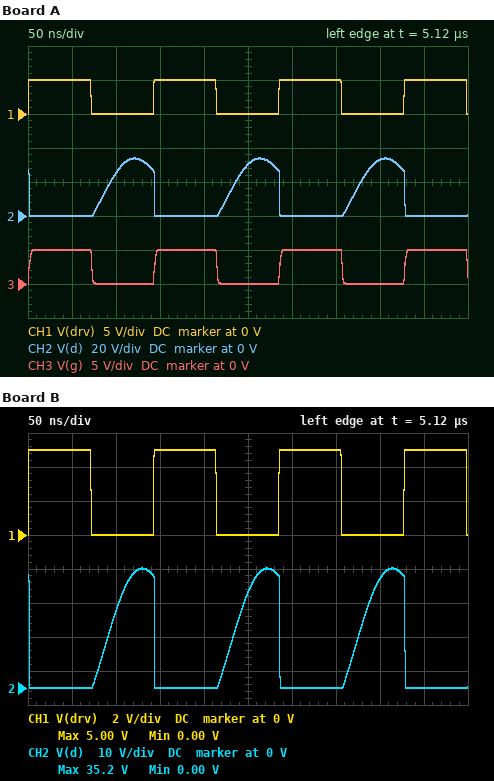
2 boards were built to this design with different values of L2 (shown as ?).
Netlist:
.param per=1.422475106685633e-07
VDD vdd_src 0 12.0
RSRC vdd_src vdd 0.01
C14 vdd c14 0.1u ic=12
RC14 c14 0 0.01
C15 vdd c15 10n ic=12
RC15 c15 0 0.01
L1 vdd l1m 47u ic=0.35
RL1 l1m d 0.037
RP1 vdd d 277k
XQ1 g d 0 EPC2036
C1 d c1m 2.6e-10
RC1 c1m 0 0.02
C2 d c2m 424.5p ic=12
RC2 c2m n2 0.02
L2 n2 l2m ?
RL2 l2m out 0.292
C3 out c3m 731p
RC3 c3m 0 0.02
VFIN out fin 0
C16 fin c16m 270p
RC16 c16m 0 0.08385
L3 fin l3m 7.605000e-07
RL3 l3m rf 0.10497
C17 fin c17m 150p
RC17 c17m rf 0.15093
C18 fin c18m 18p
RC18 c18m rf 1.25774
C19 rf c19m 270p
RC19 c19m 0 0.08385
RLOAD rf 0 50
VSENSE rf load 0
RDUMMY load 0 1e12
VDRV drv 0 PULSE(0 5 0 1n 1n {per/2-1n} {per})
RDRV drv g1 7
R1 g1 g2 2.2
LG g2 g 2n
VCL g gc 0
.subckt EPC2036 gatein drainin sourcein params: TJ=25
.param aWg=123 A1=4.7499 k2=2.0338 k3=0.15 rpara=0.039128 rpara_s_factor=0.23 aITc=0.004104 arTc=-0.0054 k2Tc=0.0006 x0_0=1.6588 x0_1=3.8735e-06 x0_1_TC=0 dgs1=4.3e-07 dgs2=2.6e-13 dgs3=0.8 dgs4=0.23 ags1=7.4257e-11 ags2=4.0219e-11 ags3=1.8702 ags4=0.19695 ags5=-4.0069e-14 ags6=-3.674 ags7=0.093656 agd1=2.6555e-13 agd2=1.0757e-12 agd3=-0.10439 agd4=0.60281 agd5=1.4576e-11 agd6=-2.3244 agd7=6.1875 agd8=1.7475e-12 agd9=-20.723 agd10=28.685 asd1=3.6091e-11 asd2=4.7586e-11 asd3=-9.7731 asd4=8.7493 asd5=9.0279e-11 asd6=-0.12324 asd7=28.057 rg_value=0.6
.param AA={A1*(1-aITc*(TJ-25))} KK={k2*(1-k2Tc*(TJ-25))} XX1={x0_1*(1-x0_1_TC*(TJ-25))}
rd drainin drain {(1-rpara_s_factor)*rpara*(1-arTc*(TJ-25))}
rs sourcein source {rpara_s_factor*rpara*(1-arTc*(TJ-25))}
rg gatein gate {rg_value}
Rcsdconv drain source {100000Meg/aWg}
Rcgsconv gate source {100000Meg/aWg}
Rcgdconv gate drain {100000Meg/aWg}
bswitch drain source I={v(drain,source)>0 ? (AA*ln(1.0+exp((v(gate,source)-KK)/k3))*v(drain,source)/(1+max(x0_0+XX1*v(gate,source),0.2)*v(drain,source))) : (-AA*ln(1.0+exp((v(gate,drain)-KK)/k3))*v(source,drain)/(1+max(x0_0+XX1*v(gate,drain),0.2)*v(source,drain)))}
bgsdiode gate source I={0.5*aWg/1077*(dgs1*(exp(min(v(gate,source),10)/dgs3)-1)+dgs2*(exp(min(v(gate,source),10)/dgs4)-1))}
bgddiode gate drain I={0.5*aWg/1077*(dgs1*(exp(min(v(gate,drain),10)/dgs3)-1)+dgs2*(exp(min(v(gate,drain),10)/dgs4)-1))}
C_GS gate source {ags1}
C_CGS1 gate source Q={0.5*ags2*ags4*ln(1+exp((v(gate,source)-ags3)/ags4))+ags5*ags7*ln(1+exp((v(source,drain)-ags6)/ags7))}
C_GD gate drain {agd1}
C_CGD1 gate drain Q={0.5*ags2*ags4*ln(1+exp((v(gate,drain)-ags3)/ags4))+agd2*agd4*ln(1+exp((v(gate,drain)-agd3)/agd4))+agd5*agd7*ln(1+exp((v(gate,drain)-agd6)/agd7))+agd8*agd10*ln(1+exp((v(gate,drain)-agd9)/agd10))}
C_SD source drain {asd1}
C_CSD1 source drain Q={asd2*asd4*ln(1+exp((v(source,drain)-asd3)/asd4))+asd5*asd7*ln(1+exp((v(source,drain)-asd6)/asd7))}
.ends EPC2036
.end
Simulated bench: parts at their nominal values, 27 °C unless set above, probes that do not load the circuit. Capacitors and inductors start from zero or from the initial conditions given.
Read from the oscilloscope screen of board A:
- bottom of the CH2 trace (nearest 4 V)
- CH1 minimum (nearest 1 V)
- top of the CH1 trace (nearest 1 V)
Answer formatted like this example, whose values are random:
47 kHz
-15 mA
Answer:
0 V
0 V
5 V
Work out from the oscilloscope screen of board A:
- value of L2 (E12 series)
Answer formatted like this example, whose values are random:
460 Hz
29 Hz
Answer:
3.3 µH
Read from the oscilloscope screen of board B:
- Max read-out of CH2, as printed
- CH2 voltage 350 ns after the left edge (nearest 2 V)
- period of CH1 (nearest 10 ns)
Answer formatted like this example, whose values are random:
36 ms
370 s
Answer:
35.2 V
0 V
140 ns
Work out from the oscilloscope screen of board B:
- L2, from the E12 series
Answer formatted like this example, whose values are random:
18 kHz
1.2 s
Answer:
3.9 µH
